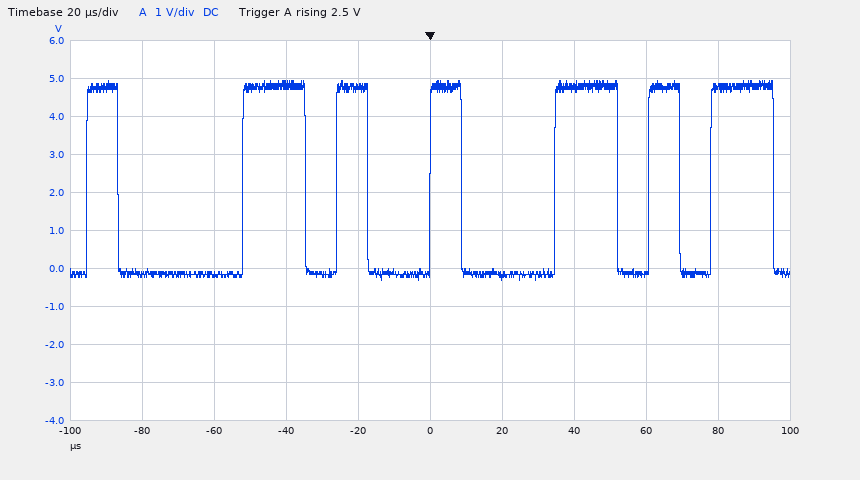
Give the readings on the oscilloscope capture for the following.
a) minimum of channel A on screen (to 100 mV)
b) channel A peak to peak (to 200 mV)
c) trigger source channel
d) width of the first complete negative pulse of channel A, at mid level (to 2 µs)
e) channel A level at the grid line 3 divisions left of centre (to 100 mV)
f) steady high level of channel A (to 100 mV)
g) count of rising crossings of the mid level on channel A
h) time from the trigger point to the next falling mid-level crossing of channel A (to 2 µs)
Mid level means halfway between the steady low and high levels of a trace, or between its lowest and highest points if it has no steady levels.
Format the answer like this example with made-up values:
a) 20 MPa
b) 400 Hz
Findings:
a) -300 mV
b) 5.2 V
c) channel A
d) 34 µs
e) -200 mV
f) 4.8 V
g) 7
h) 8 µs
